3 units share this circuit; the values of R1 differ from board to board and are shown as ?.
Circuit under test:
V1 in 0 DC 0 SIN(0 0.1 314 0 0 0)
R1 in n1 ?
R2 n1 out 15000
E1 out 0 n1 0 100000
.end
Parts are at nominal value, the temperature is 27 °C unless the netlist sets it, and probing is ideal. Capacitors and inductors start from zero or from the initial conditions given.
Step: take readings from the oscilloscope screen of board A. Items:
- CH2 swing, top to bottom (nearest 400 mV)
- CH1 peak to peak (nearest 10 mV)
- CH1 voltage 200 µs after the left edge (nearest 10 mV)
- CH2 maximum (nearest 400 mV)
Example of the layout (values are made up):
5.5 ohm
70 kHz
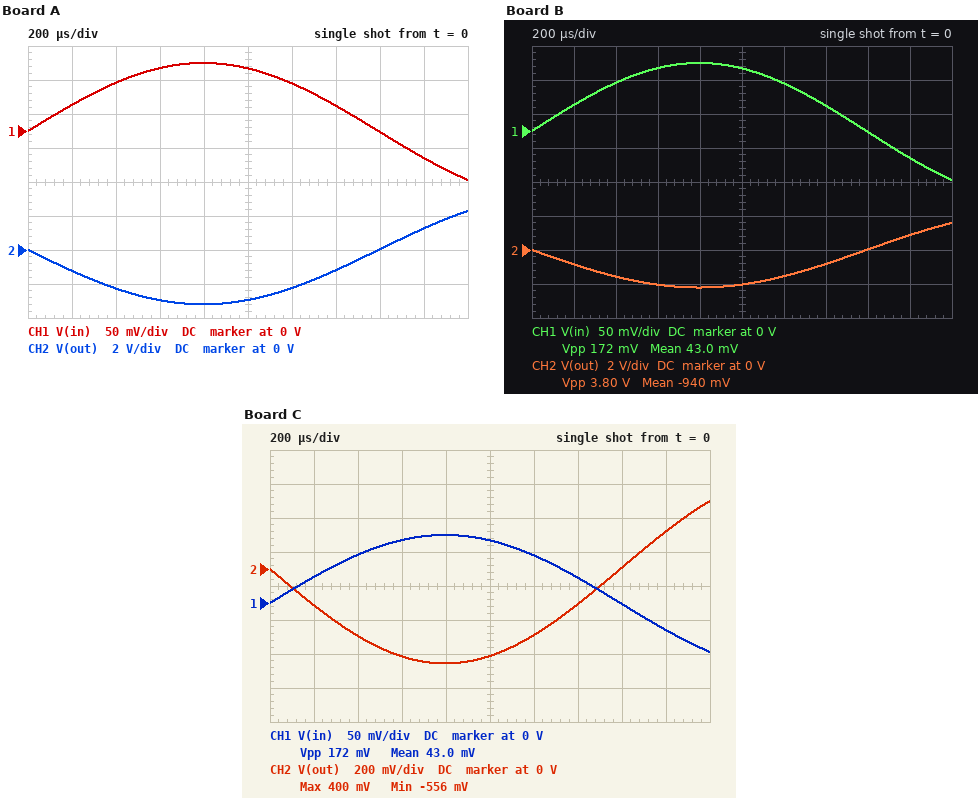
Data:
5.6 V
170 mV
40 mV
2.4 V
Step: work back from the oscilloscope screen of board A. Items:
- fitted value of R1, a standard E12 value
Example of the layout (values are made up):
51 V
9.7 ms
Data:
470 Ω
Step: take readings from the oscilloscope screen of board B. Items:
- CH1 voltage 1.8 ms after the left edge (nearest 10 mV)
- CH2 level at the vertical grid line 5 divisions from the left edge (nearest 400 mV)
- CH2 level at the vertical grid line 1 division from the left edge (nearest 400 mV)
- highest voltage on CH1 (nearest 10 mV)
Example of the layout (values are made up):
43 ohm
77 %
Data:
-40 mV
-2.0 V
-800 mV
100 mV
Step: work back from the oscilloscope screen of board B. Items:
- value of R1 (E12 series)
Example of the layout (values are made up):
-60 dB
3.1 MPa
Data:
680 Ω
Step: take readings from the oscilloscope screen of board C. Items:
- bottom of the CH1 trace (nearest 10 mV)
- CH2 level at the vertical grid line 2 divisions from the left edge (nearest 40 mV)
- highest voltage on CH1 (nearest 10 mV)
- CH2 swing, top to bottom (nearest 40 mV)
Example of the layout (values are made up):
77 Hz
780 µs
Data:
-70 mV
-400 mV
100 mV
960 mV
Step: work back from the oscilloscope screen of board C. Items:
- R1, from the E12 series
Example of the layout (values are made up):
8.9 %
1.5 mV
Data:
2.7 kΩ
